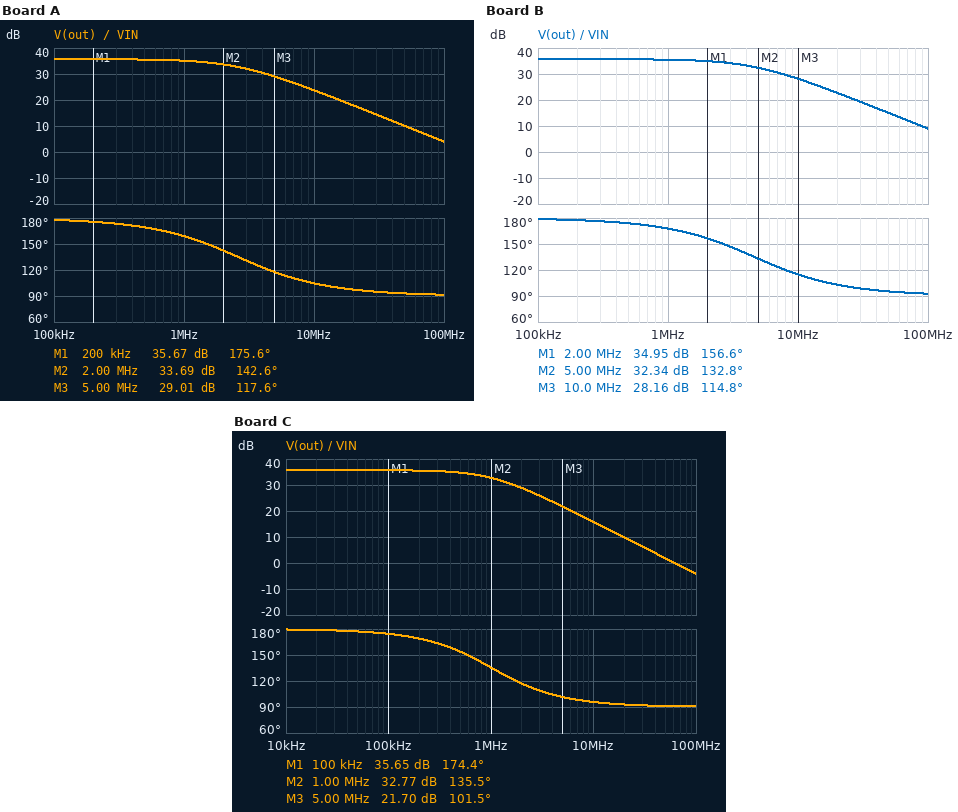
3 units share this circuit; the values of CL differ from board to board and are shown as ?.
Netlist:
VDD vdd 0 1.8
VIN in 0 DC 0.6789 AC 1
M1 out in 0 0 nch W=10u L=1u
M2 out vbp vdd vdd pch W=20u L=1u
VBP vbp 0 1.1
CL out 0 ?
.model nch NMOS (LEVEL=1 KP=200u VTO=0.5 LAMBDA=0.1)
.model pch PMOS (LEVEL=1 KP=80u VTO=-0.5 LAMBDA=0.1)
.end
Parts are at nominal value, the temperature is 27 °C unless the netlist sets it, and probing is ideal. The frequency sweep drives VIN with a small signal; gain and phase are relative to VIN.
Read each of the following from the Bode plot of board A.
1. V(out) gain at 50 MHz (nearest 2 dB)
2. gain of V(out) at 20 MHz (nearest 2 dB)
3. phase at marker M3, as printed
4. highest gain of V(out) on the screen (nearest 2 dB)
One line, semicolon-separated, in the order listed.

10 dB; 18 dB; 117.6 deg; 36 dB
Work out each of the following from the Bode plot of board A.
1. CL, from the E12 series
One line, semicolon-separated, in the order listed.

390 fF
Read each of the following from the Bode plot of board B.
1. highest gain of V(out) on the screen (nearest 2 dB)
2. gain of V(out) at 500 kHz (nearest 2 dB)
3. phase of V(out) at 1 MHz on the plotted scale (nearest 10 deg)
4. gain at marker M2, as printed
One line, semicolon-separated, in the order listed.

36 dB; 36 dB; 170 deg; 32.34 dB
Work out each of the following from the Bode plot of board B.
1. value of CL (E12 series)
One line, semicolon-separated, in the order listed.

220 fF
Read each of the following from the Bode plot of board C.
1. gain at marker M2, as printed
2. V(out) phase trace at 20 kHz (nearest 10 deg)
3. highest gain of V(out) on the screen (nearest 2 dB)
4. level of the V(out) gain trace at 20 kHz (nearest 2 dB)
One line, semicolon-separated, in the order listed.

32.77 dB; 180 deg; 36 dB; 36 dB
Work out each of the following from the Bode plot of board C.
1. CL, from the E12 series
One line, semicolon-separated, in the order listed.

1 pF
